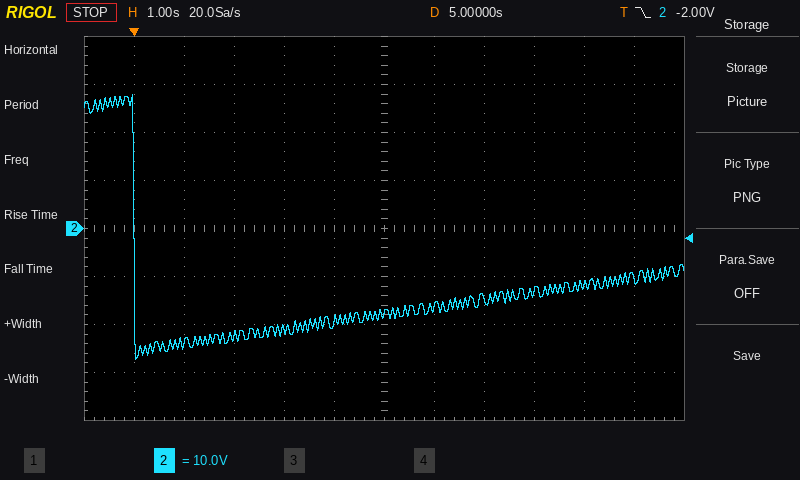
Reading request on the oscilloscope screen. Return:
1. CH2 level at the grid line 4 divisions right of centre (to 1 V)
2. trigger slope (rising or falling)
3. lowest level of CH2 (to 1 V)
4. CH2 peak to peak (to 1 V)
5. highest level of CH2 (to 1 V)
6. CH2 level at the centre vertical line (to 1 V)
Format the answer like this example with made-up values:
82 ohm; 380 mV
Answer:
-12 V; falling; -27 V; 55 V; 28 V; -18 V
